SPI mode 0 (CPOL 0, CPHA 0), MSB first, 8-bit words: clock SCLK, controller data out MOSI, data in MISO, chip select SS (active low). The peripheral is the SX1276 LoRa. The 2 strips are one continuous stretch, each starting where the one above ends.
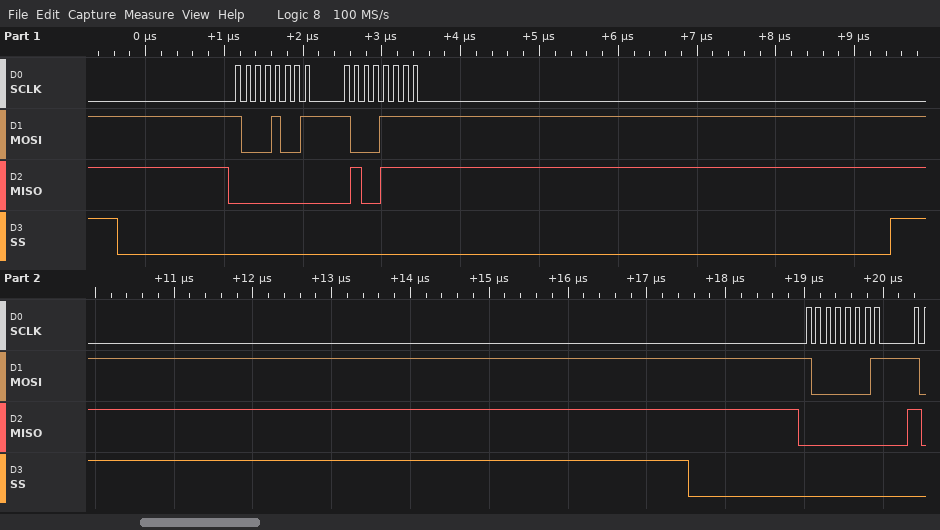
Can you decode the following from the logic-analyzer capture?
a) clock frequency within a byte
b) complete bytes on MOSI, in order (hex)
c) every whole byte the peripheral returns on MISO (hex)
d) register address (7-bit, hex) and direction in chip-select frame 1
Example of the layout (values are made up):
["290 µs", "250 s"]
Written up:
["8 MHz", "89 8F 81", "00 4F 00", "0x09 write"]
